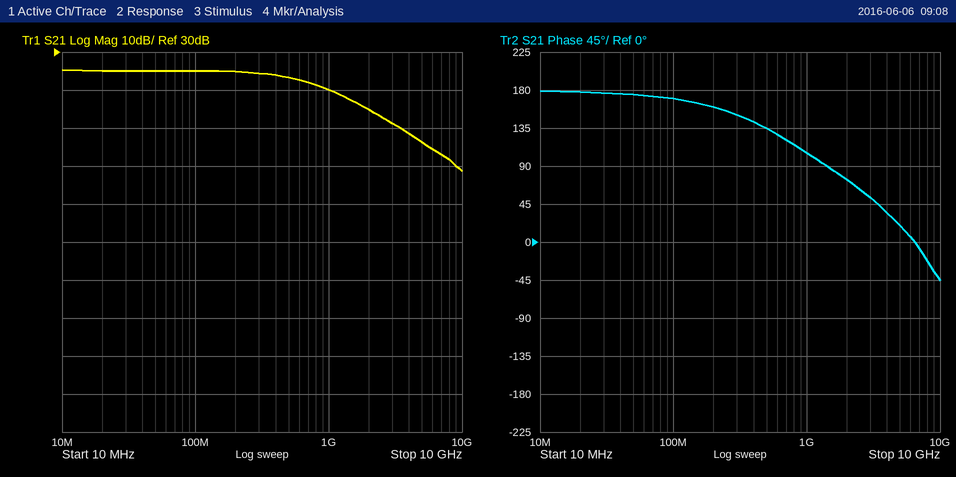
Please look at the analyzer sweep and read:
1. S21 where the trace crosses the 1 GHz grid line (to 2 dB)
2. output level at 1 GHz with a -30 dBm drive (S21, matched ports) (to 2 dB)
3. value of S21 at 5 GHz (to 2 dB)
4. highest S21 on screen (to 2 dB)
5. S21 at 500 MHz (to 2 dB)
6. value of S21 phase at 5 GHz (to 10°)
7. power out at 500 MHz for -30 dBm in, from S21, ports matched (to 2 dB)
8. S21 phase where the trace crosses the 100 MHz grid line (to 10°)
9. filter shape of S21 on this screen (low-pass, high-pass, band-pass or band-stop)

20 dB
-10 dBm
6 dB
26 dB
24 dB
20°
-6 dBm
170°
low-pass
